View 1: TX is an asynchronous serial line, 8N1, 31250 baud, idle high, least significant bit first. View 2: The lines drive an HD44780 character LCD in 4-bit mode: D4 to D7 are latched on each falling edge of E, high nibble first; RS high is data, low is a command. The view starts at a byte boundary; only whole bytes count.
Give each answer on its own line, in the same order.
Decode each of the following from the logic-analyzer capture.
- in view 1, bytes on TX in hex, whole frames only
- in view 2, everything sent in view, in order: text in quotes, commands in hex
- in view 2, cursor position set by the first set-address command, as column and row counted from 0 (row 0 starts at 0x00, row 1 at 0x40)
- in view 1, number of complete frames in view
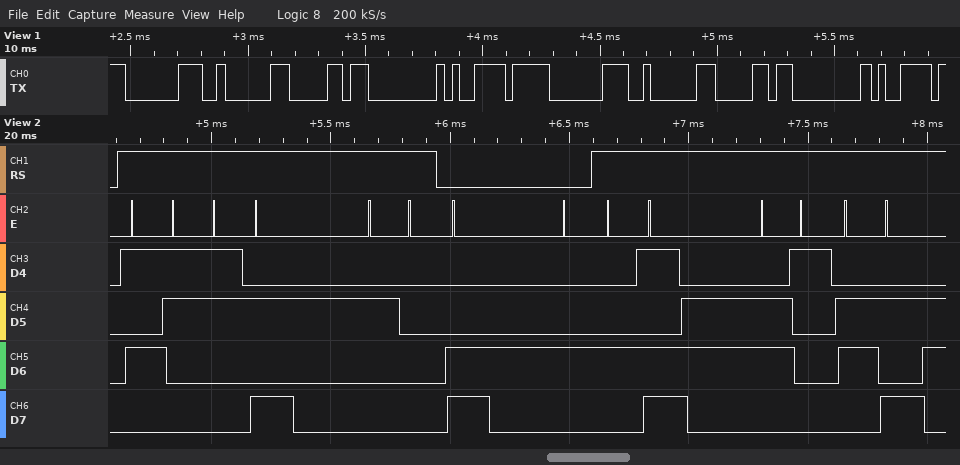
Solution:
0xC0 0x02 0xB0 0x00 0x79 0xC0 0x02 0xB0 0x00 0x79
"S: " 0xC4 "Maj"
column 4, row 1
10
